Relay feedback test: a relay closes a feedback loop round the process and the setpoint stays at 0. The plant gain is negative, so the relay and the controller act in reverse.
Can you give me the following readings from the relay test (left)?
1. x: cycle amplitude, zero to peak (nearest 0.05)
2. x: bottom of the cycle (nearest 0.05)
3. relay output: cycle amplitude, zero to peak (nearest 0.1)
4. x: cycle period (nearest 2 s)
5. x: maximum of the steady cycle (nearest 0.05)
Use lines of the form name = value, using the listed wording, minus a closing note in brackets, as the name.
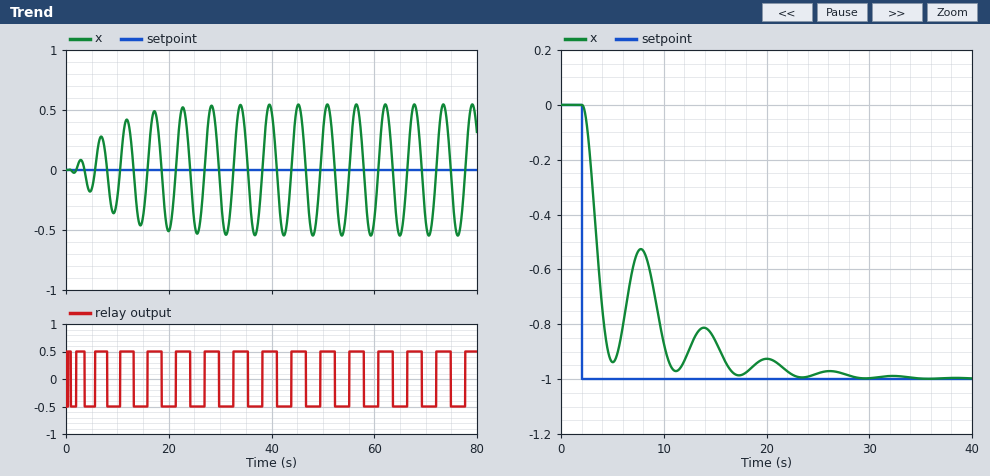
x: cycle amplitude, zero to peak = 0.55
x: bottom of the cycle = -0.55
relay output: cycle amplitude, zero to peak = 0.5
x: cycle period = 6 s
x: maximum of the steady cycle = 0.55
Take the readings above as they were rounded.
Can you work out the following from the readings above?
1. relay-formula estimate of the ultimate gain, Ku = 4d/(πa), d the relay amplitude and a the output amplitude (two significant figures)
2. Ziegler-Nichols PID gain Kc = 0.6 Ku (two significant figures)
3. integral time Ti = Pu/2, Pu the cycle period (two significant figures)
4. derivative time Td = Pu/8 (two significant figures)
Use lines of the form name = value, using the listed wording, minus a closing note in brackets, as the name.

relay-formula estimate of the ultimate gain, Ku = 4d/(πa), d the relay amplitude and a the output amplitude = 1.2
Ziegler-Nichols PID gain Kc = 0.6 Ku = 0.72
integral time Ti = Pu/2, Pu the cycle period = 3.0 s
derivative time Td = Pu/8 = 0.75 s
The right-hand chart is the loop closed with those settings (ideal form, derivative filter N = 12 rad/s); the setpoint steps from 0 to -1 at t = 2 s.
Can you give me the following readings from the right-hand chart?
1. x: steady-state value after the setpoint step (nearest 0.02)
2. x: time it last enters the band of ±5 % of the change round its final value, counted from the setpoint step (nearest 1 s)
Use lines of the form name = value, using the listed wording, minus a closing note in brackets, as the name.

x: steady-state value after the setpoint step = -1.00
x: time it last enters the band of ±5 % of the change round its final value, counted from the setpoint step = 19 s
